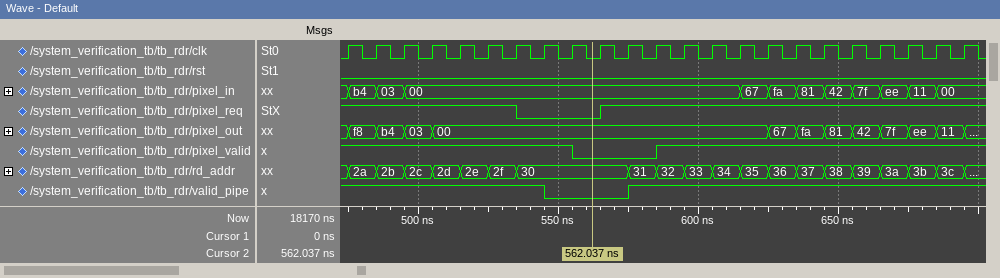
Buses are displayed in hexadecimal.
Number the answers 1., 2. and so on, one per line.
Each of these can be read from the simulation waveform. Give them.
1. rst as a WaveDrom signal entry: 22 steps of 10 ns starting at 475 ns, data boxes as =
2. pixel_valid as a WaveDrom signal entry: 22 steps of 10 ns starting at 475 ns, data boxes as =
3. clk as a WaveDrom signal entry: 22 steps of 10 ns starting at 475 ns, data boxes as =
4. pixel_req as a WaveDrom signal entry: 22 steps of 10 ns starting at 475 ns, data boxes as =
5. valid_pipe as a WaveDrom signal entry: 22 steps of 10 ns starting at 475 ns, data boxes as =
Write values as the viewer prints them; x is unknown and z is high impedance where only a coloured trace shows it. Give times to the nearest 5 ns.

1. {name: 'rst', wave: '0.....................'}
2. {name: 'pixel_valid', wave: '1.......0..1..........'}
3. {name: 'clk', wave: 'p.....................'}
4. {name: 'pixel_req', wave: '1.....0..1............'}
5. {name: 'valid_pipe', wave: '1......0..1...........'}
